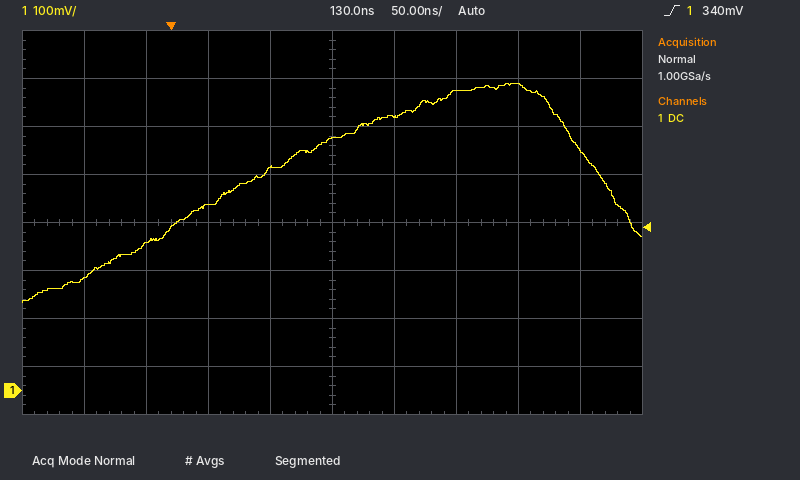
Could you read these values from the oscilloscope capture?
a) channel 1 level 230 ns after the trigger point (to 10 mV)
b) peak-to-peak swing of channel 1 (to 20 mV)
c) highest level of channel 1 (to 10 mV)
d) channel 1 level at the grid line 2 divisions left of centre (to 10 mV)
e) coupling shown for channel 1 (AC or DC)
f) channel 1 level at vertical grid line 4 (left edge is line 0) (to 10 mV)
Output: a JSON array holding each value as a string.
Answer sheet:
["620 mV", "460 mV", "640 mV", "390 mV", "DC", "460 mV"]
